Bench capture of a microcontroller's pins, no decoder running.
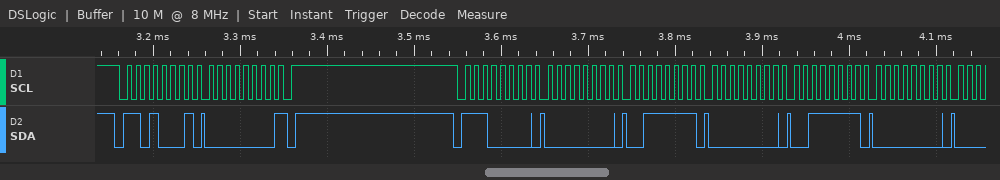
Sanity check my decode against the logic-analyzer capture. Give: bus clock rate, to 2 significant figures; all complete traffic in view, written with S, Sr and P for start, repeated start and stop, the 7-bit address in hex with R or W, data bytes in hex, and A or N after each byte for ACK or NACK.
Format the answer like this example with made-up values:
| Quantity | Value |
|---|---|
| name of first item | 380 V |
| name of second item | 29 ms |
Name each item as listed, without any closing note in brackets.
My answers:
| Quantity | Value |
|---|---|
| bus clock rate, to 2 significant figures | 100 kHz |
| all complete traffic in view, written with S, Sr and P for start, repeated start and stop, the 7-bit address in hex with R or W, data bytes in hex, and A or N after each byte for ACK or NACK | S 68R A 00 N P S 70W A 00 A 3F A 00 A 3F A 00 A |
